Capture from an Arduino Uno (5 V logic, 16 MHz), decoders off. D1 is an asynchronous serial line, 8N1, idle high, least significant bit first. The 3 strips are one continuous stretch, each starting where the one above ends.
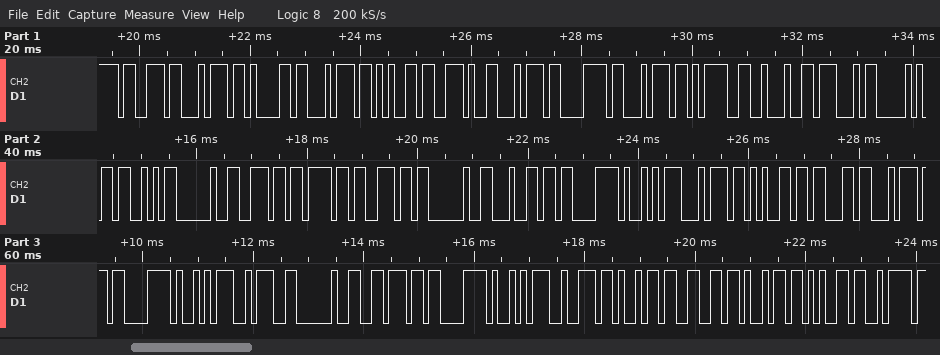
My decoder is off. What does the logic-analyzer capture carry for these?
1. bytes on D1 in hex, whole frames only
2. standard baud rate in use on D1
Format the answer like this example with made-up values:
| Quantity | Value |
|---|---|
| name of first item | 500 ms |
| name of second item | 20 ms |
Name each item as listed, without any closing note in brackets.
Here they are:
| Quantity | Value |
|---|---|
| bytes on D1 in hex, whole frames only | 73 74 61 74 65 2E 74 78 74 3D 22 47 50 53 20 6E 6F 6E 20 64 C3 A9 74 65 63 74 C3 A9 3A 20 76 C3 A9 72 69 66 69 65 7A |
| standard baud rate in use on D1 | 9600 baud |
